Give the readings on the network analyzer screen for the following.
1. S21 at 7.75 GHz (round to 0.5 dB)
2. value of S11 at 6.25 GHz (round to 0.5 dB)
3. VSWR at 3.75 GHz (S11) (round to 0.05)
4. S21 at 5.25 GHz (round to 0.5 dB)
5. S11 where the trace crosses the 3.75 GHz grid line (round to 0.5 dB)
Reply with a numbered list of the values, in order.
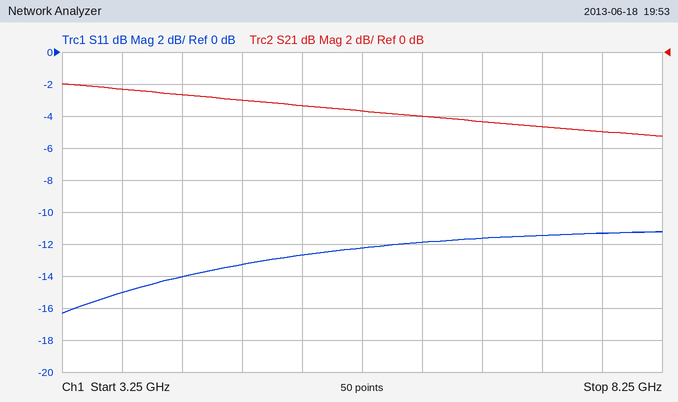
1. -5.0 dB
2. -12.0 dB
3. 1.45
4. -3.5 dB
5. -15.0 dB
